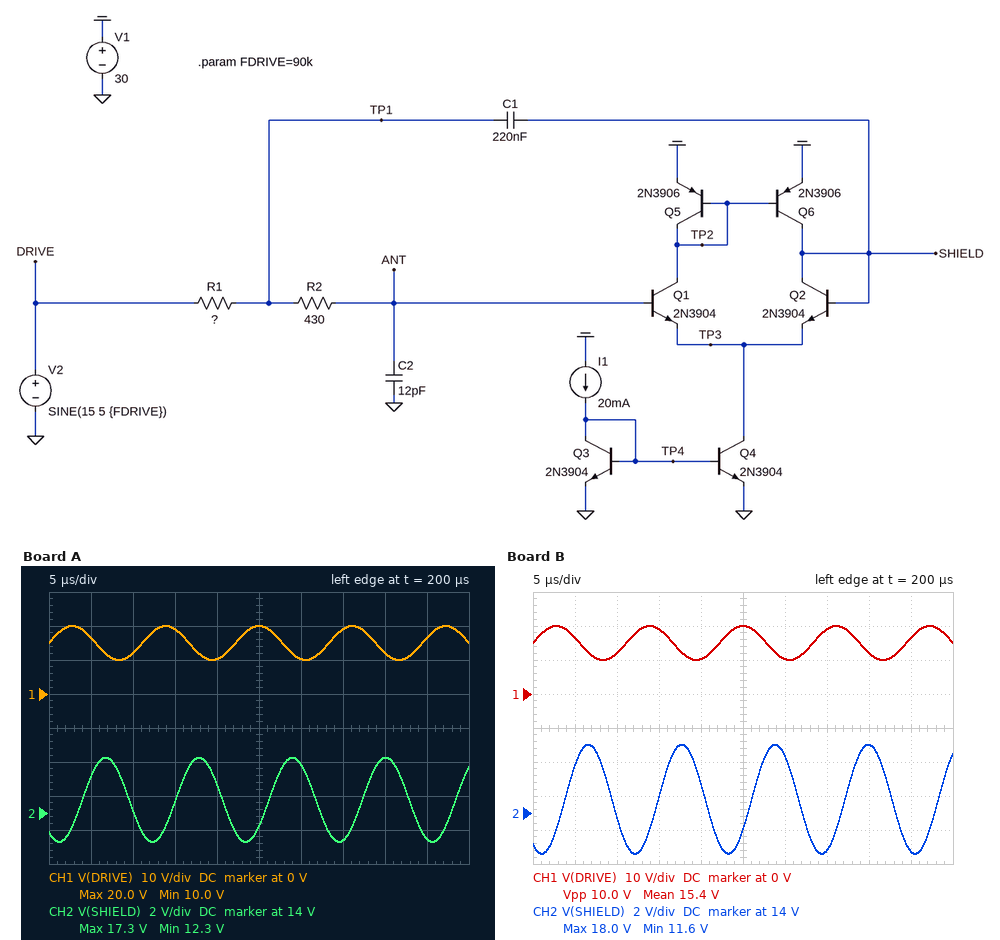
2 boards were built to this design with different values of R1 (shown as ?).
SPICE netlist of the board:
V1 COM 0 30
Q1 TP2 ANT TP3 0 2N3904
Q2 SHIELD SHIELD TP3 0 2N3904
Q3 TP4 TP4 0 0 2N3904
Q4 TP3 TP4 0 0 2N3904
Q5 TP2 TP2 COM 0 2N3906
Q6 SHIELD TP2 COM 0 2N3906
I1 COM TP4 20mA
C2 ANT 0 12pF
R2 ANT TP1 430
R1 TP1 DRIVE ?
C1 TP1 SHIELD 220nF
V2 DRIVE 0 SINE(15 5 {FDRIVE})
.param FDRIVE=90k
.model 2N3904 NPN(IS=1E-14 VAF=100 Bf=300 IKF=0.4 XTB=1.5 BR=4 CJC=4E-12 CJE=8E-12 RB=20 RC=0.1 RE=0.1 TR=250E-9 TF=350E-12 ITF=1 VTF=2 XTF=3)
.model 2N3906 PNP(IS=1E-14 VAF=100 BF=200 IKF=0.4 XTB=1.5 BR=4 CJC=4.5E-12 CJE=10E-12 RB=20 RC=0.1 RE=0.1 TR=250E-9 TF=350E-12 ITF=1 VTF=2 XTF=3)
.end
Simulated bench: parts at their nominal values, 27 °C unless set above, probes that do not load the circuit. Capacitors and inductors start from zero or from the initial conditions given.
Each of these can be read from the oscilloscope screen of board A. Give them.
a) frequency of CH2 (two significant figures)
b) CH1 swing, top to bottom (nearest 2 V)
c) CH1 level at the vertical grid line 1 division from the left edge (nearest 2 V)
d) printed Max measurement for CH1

90 kHz
10 V
16 V
20.0 V
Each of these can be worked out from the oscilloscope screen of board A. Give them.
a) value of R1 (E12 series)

6.8 kΩ
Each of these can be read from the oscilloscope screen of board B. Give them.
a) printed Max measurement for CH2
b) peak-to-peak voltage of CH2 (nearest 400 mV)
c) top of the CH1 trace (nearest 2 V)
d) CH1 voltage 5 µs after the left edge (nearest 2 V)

18.0 V
6.4 V
20 V
16 V
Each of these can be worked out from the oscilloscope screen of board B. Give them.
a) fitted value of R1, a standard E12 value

5.6 kΩ
